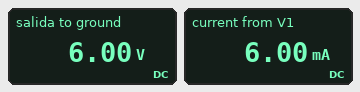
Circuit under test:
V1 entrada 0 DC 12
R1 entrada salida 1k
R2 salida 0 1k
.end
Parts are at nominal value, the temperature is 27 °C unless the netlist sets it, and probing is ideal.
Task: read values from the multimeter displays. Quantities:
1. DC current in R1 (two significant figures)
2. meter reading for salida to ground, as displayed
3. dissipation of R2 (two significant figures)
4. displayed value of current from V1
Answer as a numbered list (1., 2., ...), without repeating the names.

1. 6.0 mA
2. 6.00 V
3. 36 mW
4. 6.00 mA
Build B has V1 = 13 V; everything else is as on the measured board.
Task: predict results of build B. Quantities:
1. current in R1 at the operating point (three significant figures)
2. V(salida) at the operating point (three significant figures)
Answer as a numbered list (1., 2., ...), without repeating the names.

1. 6.50 mA
2. 6.50 V
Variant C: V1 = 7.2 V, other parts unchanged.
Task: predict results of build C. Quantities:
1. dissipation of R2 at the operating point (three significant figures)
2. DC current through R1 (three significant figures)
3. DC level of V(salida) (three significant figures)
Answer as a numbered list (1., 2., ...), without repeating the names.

1. 13.0 mW
2. 3.60 mA
3. 3.60 V
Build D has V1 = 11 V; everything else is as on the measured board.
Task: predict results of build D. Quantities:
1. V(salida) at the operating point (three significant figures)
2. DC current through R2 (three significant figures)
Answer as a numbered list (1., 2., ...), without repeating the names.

1. 5.50 V
2. 5.50 mA
